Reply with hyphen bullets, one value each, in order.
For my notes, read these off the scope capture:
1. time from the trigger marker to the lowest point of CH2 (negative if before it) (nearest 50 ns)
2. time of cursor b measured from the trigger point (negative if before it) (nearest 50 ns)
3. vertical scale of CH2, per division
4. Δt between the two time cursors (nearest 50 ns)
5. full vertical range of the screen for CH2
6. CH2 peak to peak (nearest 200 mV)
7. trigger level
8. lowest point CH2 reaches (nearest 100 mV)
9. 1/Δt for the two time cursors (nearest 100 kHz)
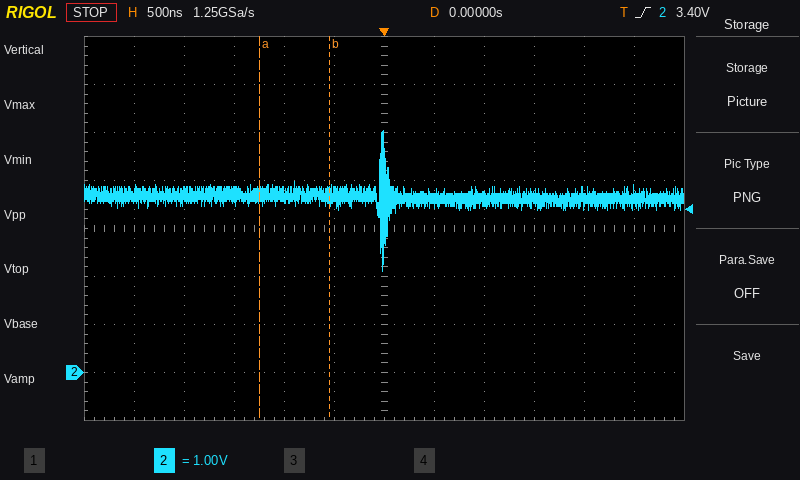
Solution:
- 0 ns
- -550 ns
- 1 V
- 700 ns
- 8 V
- 3.0 V
- 3.40 V
- 2.1 V
- 1.4 MHz
